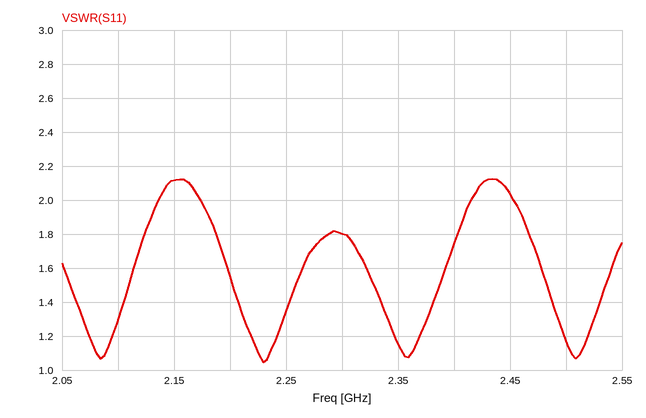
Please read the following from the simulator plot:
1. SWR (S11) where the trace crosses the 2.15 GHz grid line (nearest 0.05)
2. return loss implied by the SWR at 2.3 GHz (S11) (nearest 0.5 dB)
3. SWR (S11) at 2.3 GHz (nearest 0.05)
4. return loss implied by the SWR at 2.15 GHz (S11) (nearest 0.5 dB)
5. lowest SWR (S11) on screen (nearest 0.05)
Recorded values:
2.10
11.0 dB
1.80
9.0 dB
1.05
